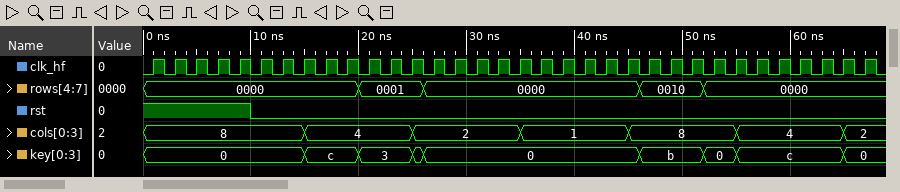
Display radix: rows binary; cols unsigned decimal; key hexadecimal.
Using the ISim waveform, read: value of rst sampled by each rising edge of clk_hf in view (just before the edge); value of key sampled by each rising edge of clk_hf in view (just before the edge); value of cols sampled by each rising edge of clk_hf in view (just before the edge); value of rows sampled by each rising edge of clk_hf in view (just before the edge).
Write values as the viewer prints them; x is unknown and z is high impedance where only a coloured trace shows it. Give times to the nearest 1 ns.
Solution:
1 1 1 1 1 0 0 0 0 0 0 0 0 0 0 0 0 0 0 0 0 0 0 0 0 0 0 0 0 0 0 0 0 0
0, 0, 0, 0, 0, 0, 0, 0, c, c, 3, 3, 3, 0, 0, 0, 0, 0, 0, 0, 0, 0, 0, b, b, b, 0, 0, c, c, c, c, c, 0
8, 8, 8, 8, 8, 8, 8, 8, 4, 4, 4, 4, 4, 2, 2, 2, 2, 2, 1, 1, 1, 1, 1, 8, 8, 8, 8, 8, 4, 4, 4, 4, 4, 2
0000, 0000, 0000, 0000, 0000, 0000, 0000, 0000, 0000, 0000, 0001, 0001, 0001, 0000, 0000, 0000, 0000, 0000, 0000, 0000, 0000, 0000, 0000, 0010, 0010, 0010, 0000, 0000, 0000, 0000, 0000, 0000, 0000, 0000
